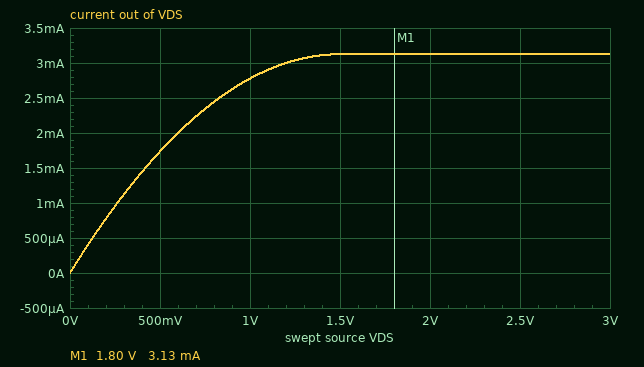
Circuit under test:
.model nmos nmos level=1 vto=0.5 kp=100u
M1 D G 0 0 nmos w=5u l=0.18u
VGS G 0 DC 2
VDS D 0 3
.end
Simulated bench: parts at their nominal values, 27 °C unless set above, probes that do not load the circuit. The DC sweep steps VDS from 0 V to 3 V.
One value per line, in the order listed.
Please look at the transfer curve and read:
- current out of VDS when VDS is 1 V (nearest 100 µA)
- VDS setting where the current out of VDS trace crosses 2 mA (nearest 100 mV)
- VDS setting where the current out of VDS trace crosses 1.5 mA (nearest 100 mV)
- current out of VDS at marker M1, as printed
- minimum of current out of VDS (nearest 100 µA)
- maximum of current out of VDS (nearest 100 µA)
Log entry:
2.8 mA
600 mV
400 mV
3.13 mA
0 A
3.1 mA
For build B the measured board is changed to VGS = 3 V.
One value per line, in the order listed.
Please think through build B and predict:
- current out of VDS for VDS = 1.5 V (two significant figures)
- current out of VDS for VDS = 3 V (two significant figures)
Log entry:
7.3 mA
8.7 mA
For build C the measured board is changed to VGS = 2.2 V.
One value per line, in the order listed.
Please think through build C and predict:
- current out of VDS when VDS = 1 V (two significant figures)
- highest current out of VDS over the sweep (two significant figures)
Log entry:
3.3 mA
4.0 mA
